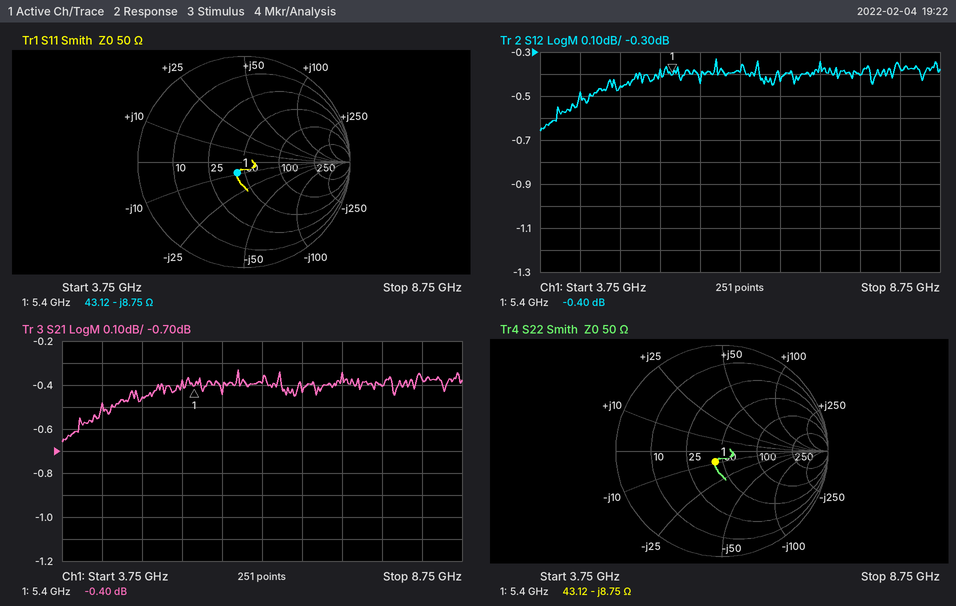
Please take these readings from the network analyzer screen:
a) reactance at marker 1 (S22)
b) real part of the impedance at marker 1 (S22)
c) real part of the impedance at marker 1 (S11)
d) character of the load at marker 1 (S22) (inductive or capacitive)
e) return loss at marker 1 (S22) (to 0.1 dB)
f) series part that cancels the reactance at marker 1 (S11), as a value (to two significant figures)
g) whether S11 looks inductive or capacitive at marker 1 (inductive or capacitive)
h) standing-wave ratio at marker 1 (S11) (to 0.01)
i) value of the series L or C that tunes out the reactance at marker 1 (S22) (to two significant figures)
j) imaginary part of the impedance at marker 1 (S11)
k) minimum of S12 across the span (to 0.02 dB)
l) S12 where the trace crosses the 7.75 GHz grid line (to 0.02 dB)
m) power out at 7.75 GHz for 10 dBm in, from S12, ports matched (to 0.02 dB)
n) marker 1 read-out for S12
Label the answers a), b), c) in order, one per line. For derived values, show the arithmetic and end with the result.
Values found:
a) -8.75 Ω
b) 43.12 Ω
c) 43.12 Ω
d) capacitive
e) 18.5 dB
f) L = 8.75 Ω/(2π × 5.4 GHz) ≈ 258 pH, so 260 pH to two significant figures
g) capacitive
h) 1.27
i) L = 8.75 Ω/(2π × 5.4 GHz) ≈ 258 pH, so 260 pH to two significant figures
j) -8.75 Ω
k) -0.66 dB
l) -0.40 dB
m) 10 dBm + (-0.40 dB) = 9.60 dBm
n) -0.40 dB
